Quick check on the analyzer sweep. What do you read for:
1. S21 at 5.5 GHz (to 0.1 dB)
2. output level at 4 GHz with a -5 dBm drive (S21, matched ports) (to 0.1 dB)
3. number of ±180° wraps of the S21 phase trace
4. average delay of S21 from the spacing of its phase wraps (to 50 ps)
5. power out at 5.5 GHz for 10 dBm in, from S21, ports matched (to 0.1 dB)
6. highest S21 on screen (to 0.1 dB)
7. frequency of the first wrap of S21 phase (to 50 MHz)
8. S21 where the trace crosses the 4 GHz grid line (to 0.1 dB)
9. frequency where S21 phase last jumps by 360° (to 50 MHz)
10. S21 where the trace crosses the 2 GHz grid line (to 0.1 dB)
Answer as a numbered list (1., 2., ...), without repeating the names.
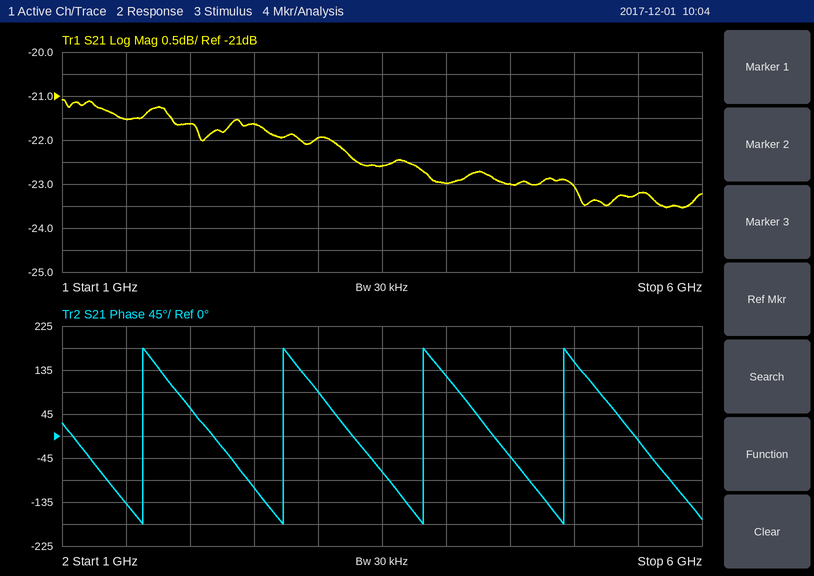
1. -23.2 dB
2. -28.0 dBm
3. 4
4. 900 ps
5. -13.2 dBm
6. -21.1 dB
7. 1.65 GHz
8. -23.0 dB
9. 4.90 GHz
10. -21.6 dB
